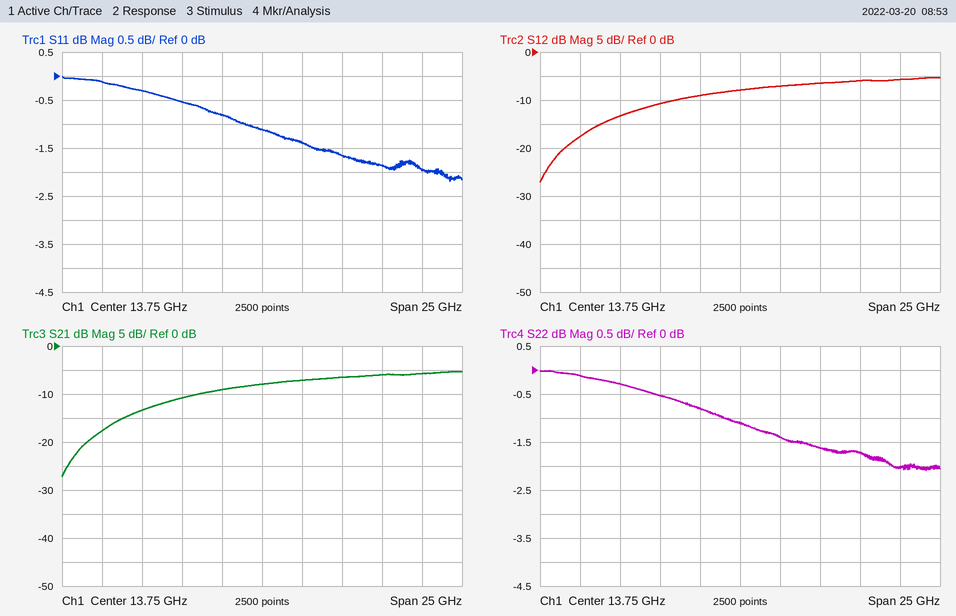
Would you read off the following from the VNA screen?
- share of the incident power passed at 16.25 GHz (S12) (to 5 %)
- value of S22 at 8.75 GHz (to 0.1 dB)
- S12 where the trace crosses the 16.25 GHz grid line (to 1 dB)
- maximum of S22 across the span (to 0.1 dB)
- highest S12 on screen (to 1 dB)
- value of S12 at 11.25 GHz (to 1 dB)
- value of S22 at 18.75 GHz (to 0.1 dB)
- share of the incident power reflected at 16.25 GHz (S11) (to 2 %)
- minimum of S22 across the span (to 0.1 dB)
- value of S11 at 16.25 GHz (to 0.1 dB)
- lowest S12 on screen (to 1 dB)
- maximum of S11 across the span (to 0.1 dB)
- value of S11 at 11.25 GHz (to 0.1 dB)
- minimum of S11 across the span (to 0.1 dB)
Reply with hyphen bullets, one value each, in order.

- 20 %
- -0.5 dB
- -7 dB
- 0.0 dB
- -5 dB
- -9 dB
- -1.6 dB
- 72 %
- -2.1 dB
- -1.4 dB
- -27 dB
- 0.0 dB
- -0.8 dB
- -2.2 dB
